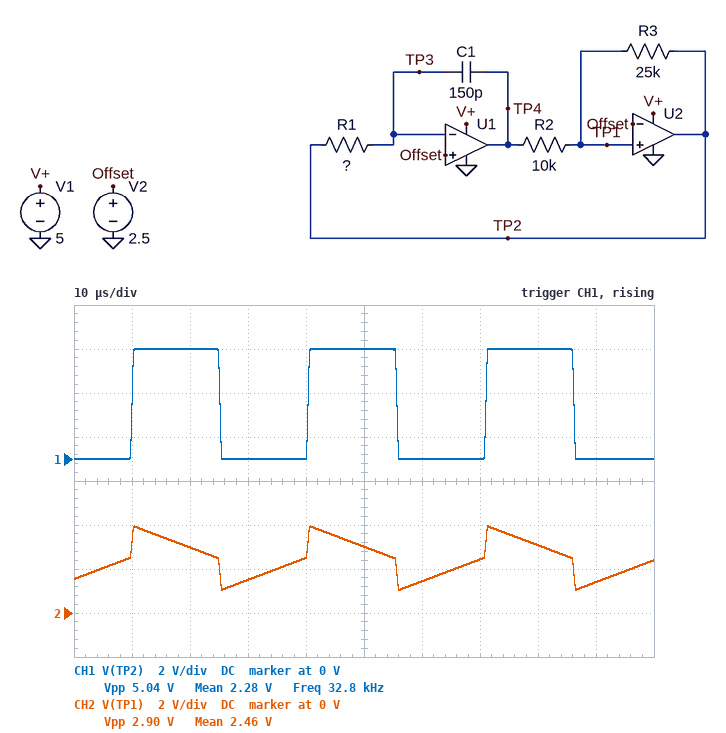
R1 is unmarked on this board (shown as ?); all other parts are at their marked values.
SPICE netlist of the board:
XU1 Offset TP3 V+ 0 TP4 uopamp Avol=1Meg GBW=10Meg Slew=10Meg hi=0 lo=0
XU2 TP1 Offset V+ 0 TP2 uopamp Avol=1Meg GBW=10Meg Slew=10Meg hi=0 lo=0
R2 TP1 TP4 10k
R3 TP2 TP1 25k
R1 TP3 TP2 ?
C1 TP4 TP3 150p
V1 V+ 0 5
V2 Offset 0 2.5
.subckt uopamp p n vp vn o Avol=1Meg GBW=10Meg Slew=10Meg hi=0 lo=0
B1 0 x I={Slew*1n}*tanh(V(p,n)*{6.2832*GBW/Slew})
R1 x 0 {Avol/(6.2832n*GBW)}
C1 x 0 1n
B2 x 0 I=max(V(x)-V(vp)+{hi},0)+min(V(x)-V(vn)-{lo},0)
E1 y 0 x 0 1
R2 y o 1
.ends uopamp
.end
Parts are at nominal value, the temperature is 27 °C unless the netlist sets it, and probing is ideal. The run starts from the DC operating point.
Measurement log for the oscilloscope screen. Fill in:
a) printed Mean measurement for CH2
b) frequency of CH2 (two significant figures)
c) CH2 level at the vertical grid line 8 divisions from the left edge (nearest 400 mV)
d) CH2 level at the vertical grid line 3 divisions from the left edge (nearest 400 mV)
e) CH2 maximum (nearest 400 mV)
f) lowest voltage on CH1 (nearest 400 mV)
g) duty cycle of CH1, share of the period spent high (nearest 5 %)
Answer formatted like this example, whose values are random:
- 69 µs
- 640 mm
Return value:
- 2.46 V
- 33 kHz
- 3.2 V
- 1.6 V
- 4.0 V
- 0 V
- 50 %
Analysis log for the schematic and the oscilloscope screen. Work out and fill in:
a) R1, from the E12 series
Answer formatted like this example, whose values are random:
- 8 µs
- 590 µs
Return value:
- 120 kΩ
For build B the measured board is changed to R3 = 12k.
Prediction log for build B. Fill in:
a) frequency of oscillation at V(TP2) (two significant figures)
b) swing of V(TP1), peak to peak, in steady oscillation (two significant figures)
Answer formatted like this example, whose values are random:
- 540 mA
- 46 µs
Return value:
- 16 kHz
- 4.6 V
